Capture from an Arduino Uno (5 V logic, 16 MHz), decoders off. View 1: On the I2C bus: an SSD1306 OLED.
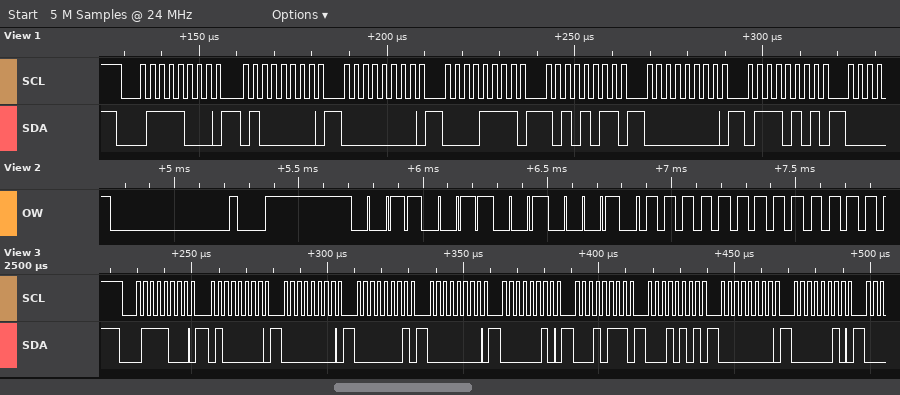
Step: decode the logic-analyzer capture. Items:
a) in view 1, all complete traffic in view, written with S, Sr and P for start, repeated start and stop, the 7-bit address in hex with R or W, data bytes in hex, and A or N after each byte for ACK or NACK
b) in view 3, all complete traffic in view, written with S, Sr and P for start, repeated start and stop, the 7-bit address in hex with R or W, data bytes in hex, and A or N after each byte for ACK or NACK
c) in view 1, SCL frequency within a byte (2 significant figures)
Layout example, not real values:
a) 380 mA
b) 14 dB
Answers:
a) S 3CW A 40 A 00 A 0F A AB A 00 A 75 A
b) S 3CW A 40 A 00 A 01 A 00 A 02 A 17 A 15 A 00 A 02 A
c) 400 kHz
